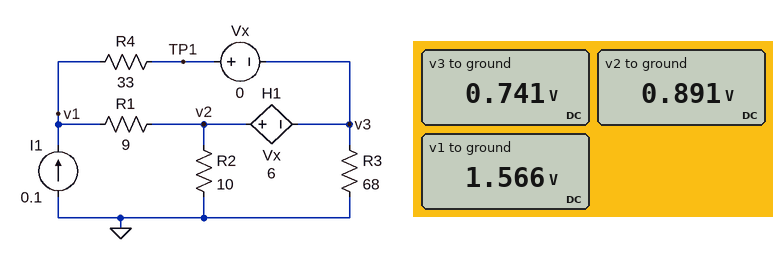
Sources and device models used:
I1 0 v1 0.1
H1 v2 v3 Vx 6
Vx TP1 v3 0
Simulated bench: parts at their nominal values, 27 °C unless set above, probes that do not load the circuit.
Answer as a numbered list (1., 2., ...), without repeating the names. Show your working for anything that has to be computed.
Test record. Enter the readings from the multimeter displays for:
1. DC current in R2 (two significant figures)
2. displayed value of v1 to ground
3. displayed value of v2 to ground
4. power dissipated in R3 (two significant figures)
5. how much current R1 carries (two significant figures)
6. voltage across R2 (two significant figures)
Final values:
1. (891 mV) / 10 Ω = 89 mA
2. 1.566 V
3. 0.891 V
4. (741 mV)^2 / 68 Ω = 8.1 mW
5. (1.566 V - 891 mV) / 9 Ω = 75 mA
6. 891 mV = 890 mV
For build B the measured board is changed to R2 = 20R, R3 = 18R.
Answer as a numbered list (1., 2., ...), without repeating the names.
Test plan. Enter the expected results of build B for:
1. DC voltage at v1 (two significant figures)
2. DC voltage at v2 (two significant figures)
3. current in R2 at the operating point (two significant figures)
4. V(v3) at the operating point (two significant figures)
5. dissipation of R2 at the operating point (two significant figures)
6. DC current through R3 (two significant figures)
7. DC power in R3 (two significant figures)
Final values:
1. 1.7 V
2. 1.0 V
3. 51 mA
4. 880 mV
5. 53 mW
6. 49 mA
7. 43 mW
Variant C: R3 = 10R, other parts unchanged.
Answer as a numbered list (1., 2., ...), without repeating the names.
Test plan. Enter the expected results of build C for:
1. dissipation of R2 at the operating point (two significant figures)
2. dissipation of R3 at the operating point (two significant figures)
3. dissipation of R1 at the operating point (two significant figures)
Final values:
1. 33 mW
2. 18 mW
3. 51 mW
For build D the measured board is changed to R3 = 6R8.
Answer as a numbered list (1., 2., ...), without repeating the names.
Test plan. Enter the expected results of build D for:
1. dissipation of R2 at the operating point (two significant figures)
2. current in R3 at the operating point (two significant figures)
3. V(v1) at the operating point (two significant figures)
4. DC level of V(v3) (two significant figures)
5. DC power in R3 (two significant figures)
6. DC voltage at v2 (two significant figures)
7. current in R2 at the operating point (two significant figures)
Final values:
1. 24 mW
2. 51 mA
3. 1.2 V
4. 340 mV
5. 17 mW
6. 490 mV
7. 49 mA
